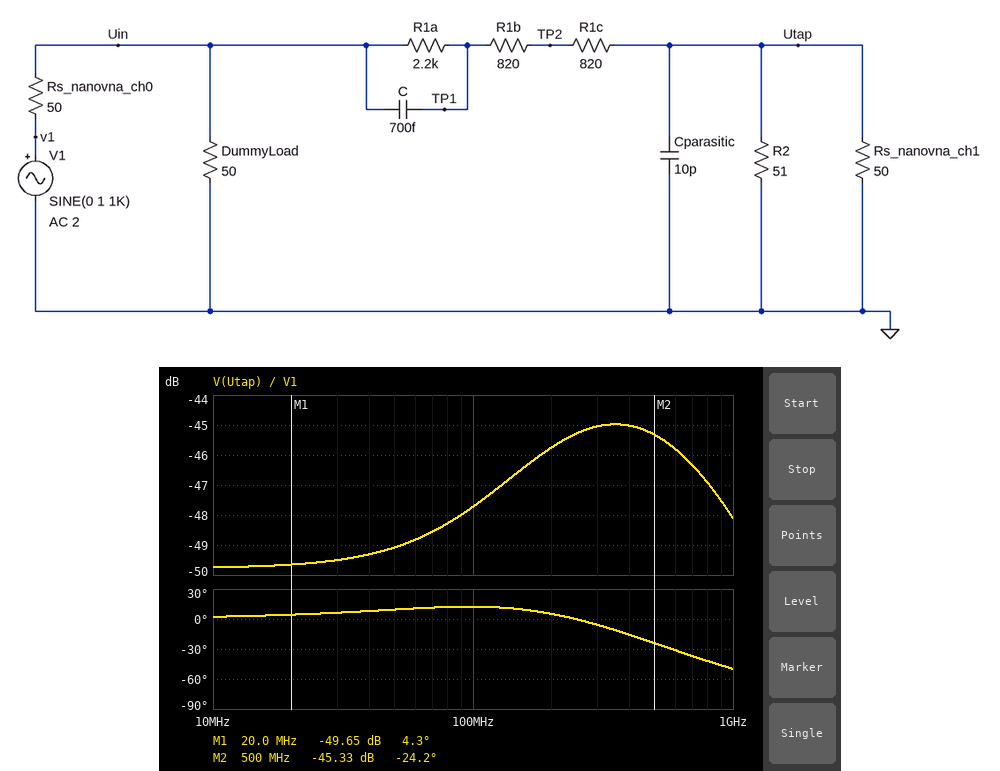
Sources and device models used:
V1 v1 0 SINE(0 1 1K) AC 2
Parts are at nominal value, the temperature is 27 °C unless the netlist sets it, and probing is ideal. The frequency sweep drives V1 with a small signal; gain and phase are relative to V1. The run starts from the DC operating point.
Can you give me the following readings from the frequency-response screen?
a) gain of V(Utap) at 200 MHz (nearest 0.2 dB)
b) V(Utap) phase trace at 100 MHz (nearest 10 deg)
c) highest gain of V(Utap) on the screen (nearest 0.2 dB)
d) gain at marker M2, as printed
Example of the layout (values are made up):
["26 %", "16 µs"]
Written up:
["-45.8 dB", "10 deg", "-45.0 dB", "-45.33 dB"]
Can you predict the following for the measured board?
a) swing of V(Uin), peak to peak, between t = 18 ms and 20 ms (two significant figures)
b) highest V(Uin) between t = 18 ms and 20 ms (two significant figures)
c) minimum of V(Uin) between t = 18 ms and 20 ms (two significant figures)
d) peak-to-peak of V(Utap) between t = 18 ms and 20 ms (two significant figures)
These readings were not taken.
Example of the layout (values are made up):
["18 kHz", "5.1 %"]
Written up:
["990 mV", "500 mV", "-500 mV", "6.5 mV"]
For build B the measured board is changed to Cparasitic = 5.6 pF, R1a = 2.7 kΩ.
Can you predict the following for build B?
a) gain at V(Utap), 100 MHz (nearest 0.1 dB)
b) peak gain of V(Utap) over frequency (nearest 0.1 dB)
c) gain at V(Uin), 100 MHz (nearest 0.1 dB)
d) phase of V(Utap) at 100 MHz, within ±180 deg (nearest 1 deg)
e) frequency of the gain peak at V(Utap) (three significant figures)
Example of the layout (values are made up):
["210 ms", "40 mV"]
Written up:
["-47.9 dB", "-43.9 dB", "-6.1 dB", "20 deg", "472 MHz"]
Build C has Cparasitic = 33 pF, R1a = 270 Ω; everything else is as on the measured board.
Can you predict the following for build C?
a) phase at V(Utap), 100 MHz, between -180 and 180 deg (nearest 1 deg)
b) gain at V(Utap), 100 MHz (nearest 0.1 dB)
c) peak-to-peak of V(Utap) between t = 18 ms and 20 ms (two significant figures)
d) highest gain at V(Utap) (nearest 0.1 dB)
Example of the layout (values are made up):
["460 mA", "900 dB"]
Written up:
["-26 deg", "-44.8 dB", "13 mV", "-43.8 dB"]
